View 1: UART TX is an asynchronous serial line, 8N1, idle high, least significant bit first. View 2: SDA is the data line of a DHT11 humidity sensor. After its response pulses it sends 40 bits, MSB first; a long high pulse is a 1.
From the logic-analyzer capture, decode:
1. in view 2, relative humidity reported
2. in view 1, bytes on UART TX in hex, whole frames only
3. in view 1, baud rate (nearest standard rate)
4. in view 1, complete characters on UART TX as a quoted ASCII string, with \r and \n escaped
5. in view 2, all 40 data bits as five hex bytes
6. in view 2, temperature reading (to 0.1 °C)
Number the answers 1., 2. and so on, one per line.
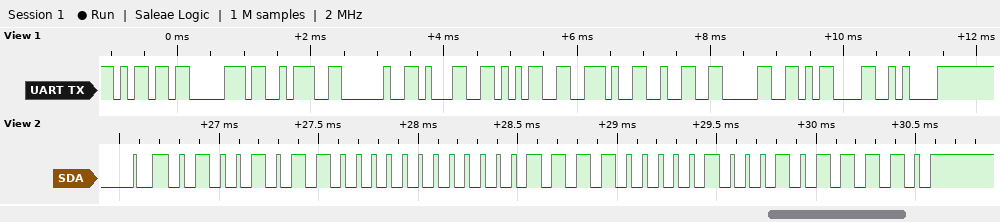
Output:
1. 75 %
2. 0x6D 0x70 0x3A 0x20 0x31 0x35 0x2E 0x32 0x30 0x0D 0x0A
3. 9600 baud
4. "mp: 15.20\r\n"
5. 4B 00 0F 04 5E
6. 15.4 °C
